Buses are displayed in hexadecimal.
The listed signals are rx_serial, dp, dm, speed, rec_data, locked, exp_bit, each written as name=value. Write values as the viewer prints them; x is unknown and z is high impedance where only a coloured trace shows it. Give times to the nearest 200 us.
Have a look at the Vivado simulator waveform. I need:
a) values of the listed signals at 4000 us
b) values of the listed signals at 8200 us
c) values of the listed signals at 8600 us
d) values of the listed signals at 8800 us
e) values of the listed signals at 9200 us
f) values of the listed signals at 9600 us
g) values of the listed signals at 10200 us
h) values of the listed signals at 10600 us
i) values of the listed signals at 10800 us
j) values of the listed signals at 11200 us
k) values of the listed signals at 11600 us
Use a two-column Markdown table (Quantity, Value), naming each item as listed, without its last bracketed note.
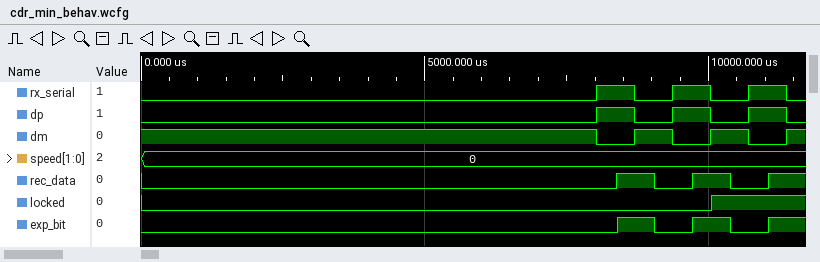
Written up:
| Quantity | Value |
|---|---|
| values of the listed signals at 4000 us | rx_serial=0, dp=0, dm=1, speed=0, rec_data=0, locked=0, exp_bit=0 |
| values of the listed signals at 8200 us | rx_serial=1, dp=1, dm=0, speed=0, rec_data=0, locked=0, exp_bit=0 |
| values of the listed signals at 8600 us | rx_serial=1, dp=1, dm=0, speed=0, rec_data=1, locked=0, exp_bit=1 |
| values of the listed signals at 8800 us | rx_serial=0, dp=0, dm=1, speed=0, rec_data=1, locked=0, exp_bit=1 |
| values of the listed signals at 9200 us | rx_serial=0, dp=0, dm=1, speed=0, rec_data=0, locked=0, exp_bit=0 |
| values of the listed signals at 9600 us | rx_serial=1, dp=1, dm=0, speed=0, rec_data=0, locked=0, exp_bit=0 |
| values of the listed signals at 10200 us | rx_serial=0, dp=0, dm=1, speed=0, rec_data=1, locked=1, exp_bit=1 |
| values of the listed signals at 10600 us | rx_serial=0, dp=0, dm=1, speed=0, rec_data=0, locked=1, exp_bit=0 |
| values of the listed signals at 10800 us | rx_serial=1, dp=1, dm=0, speed=0, rec_data=0, locked=1, exp_bit=0 |
| values of the listed signals at 11200 us | rx_serial=1, dp=1, dm=0, speed=0, rec_data=1, locked=1, exp_bit=1 |
| values of the listed signals at 11600 us | rx_serial=0, dp=0, dm=1, speed=0, rec_data=1, locked=1, exp_bit=1 |
